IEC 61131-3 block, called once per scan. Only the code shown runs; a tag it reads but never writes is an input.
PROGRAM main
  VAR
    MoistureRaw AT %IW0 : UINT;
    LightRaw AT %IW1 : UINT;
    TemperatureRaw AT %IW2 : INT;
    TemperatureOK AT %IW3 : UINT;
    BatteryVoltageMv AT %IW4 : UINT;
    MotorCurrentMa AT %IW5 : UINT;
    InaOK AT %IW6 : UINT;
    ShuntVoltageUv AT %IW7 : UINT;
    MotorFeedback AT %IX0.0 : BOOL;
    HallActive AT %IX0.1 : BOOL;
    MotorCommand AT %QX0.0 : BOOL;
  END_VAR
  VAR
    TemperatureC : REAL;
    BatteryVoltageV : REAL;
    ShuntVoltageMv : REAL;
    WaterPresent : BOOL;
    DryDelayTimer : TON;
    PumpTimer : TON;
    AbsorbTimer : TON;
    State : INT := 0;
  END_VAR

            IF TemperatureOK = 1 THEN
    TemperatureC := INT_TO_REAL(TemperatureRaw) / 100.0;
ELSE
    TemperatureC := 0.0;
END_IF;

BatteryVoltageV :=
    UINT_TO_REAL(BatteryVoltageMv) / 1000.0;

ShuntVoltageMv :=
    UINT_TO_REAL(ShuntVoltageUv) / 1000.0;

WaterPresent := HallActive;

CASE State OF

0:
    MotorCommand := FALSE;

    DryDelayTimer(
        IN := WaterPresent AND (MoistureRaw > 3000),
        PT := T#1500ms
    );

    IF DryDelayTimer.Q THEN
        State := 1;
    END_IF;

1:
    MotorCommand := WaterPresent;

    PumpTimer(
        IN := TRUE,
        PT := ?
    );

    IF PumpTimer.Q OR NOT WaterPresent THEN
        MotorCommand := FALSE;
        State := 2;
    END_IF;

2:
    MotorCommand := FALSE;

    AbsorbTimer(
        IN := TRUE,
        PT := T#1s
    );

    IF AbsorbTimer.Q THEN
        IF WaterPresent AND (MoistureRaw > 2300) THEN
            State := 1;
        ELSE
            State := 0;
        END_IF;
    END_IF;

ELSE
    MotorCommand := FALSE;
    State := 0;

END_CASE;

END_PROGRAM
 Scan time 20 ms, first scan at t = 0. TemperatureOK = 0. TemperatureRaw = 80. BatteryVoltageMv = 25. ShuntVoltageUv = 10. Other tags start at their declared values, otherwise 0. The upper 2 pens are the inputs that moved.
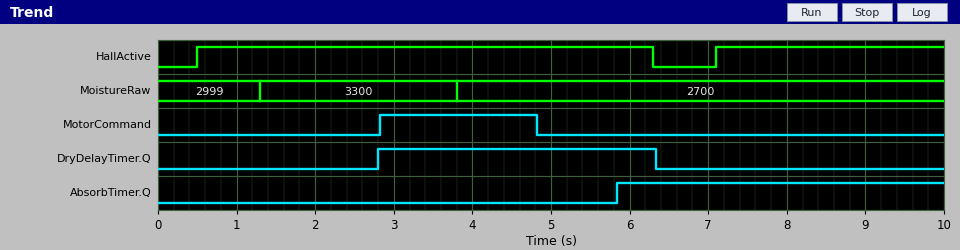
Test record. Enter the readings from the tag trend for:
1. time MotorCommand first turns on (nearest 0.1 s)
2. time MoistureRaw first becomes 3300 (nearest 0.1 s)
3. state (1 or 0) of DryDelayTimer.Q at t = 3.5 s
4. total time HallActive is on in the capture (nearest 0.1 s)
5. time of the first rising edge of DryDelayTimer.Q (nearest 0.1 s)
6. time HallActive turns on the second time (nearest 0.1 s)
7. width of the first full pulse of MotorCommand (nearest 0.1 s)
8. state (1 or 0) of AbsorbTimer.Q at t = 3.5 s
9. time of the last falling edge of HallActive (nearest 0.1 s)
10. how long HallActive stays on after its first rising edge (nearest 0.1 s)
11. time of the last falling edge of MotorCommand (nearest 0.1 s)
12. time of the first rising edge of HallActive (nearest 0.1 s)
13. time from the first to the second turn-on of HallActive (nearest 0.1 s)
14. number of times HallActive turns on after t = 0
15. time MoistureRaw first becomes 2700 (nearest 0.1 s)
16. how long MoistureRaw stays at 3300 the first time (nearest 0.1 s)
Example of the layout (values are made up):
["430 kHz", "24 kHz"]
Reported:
["2.8 s", "1.3 s", "1", "8.7 s", "2.8 s", "7.1 s", "2.0 s", "0", "6.3 s", "5.8 s", "4.8 s", "0.5 s", "6.6 s", "2", "3.8 s", "2.5 s"]
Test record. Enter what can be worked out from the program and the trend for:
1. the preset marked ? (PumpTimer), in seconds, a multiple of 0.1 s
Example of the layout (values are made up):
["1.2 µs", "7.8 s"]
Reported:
["2.0 s"]
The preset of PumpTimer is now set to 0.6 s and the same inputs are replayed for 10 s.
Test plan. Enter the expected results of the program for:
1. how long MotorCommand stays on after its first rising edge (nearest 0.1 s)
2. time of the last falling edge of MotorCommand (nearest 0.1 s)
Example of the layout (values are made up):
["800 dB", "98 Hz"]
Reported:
["0.6 s", "3.4 s"]
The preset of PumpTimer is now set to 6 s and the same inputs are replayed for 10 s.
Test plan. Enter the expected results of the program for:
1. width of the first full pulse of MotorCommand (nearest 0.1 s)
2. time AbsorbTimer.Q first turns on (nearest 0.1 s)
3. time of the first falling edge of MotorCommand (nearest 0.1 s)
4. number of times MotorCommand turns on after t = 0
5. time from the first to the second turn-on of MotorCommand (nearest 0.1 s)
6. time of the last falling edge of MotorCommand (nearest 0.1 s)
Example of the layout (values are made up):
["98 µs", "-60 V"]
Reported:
["3.5 s", "7.3 s", "6.3 s", "2", "4.5 s", "8.8 s"]
